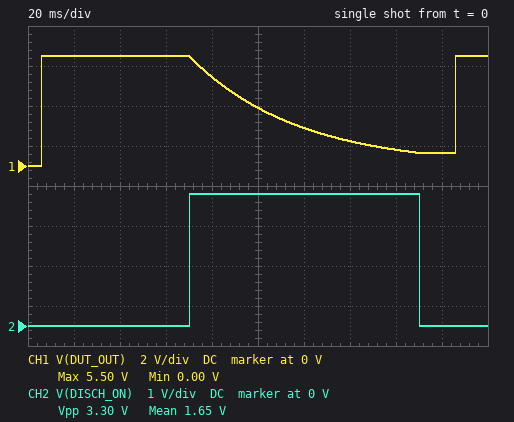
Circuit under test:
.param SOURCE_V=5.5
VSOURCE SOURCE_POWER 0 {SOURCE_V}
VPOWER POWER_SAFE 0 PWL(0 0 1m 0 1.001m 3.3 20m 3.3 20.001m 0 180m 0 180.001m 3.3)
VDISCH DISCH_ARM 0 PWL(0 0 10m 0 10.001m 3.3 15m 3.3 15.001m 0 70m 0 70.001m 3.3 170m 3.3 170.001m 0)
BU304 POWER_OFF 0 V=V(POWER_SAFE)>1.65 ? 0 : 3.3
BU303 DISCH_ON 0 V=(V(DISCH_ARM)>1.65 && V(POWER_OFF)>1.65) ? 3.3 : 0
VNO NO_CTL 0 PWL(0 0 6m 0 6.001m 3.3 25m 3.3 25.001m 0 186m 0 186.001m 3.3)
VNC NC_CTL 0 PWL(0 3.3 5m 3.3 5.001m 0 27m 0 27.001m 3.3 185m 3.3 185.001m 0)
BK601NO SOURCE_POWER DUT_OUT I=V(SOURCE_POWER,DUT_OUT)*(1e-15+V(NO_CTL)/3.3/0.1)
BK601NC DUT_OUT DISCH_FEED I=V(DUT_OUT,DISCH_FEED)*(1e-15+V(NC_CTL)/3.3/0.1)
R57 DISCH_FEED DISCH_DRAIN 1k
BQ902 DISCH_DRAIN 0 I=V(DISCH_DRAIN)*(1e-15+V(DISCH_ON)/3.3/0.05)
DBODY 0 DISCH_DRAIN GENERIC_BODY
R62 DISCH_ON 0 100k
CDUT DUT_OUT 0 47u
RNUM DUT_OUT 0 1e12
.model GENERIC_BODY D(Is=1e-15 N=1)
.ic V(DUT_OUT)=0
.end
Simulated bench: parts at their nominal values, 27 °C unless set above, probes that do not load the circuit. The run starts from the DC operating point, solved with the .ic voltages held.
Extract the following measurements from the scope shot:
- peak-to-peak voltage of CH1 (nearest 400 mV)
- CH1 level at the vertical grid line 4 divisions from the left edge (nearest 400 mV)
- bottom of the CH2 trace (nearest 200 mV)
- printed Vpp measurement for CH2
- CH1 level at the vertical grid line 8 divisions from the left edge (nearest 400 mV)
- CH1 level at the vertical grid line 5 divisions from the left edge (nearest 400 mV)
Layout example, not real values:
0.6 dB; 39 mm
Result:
5.6 V; 4.4 V; 0 V; 3.30 V; 800 mV; 2.8 V
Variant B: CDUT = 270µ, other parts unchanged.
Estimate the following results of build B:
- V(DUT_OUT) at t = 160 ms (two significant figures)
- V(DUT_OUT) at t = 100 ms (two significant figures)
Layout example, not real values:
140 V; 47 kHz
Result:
3.9 V; 4.9 V
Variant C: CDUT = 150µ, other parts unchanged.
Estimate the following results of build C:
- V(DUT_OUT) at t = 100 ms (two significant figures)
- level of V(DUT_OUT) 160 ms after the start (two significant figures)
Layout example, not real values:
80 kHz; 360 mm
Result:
4.5 V; 3.0 V
